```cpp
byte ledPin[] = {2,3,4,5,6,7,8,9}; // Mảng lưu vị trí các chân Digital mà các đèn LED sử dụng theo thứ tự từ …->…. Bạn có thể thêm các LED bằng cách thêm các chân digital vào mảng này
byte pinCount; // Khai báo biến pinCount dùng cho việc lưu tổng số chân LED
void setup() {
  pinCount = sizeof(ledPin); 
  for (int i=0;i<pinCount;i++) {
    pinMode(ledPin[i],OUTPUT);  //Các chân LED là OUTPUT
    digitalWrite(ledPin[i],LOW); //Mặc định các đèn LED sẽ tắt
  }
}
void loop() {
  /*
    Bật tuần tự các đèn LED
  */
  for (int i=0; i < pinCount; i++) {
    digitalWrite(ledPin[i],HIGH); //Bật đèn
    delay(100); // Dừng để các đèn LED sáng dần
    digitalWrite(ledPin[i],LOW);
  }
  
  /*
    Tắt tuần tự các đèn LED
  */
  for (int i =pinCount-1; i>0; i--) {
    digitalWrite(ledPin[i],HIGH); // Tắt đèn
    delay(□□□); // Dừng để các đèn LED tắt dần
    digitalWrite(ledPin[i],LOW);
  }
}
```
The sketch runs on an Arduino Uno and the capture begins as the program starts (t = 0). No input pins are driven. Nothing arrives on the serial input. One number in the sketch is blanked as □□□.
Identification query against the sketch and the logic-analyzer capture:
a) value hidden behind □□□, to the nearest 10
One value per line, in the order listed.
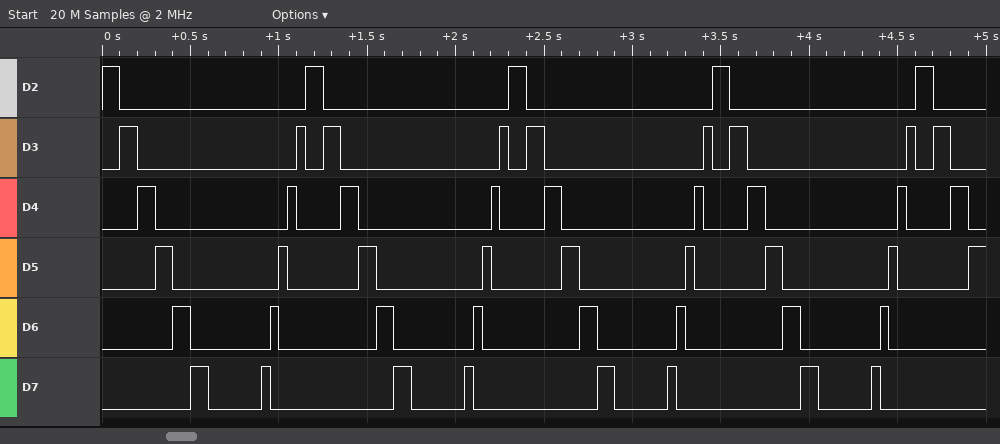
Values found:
50
